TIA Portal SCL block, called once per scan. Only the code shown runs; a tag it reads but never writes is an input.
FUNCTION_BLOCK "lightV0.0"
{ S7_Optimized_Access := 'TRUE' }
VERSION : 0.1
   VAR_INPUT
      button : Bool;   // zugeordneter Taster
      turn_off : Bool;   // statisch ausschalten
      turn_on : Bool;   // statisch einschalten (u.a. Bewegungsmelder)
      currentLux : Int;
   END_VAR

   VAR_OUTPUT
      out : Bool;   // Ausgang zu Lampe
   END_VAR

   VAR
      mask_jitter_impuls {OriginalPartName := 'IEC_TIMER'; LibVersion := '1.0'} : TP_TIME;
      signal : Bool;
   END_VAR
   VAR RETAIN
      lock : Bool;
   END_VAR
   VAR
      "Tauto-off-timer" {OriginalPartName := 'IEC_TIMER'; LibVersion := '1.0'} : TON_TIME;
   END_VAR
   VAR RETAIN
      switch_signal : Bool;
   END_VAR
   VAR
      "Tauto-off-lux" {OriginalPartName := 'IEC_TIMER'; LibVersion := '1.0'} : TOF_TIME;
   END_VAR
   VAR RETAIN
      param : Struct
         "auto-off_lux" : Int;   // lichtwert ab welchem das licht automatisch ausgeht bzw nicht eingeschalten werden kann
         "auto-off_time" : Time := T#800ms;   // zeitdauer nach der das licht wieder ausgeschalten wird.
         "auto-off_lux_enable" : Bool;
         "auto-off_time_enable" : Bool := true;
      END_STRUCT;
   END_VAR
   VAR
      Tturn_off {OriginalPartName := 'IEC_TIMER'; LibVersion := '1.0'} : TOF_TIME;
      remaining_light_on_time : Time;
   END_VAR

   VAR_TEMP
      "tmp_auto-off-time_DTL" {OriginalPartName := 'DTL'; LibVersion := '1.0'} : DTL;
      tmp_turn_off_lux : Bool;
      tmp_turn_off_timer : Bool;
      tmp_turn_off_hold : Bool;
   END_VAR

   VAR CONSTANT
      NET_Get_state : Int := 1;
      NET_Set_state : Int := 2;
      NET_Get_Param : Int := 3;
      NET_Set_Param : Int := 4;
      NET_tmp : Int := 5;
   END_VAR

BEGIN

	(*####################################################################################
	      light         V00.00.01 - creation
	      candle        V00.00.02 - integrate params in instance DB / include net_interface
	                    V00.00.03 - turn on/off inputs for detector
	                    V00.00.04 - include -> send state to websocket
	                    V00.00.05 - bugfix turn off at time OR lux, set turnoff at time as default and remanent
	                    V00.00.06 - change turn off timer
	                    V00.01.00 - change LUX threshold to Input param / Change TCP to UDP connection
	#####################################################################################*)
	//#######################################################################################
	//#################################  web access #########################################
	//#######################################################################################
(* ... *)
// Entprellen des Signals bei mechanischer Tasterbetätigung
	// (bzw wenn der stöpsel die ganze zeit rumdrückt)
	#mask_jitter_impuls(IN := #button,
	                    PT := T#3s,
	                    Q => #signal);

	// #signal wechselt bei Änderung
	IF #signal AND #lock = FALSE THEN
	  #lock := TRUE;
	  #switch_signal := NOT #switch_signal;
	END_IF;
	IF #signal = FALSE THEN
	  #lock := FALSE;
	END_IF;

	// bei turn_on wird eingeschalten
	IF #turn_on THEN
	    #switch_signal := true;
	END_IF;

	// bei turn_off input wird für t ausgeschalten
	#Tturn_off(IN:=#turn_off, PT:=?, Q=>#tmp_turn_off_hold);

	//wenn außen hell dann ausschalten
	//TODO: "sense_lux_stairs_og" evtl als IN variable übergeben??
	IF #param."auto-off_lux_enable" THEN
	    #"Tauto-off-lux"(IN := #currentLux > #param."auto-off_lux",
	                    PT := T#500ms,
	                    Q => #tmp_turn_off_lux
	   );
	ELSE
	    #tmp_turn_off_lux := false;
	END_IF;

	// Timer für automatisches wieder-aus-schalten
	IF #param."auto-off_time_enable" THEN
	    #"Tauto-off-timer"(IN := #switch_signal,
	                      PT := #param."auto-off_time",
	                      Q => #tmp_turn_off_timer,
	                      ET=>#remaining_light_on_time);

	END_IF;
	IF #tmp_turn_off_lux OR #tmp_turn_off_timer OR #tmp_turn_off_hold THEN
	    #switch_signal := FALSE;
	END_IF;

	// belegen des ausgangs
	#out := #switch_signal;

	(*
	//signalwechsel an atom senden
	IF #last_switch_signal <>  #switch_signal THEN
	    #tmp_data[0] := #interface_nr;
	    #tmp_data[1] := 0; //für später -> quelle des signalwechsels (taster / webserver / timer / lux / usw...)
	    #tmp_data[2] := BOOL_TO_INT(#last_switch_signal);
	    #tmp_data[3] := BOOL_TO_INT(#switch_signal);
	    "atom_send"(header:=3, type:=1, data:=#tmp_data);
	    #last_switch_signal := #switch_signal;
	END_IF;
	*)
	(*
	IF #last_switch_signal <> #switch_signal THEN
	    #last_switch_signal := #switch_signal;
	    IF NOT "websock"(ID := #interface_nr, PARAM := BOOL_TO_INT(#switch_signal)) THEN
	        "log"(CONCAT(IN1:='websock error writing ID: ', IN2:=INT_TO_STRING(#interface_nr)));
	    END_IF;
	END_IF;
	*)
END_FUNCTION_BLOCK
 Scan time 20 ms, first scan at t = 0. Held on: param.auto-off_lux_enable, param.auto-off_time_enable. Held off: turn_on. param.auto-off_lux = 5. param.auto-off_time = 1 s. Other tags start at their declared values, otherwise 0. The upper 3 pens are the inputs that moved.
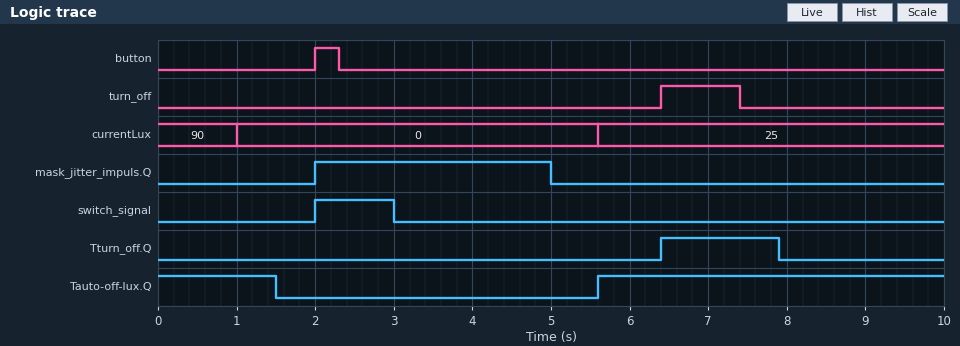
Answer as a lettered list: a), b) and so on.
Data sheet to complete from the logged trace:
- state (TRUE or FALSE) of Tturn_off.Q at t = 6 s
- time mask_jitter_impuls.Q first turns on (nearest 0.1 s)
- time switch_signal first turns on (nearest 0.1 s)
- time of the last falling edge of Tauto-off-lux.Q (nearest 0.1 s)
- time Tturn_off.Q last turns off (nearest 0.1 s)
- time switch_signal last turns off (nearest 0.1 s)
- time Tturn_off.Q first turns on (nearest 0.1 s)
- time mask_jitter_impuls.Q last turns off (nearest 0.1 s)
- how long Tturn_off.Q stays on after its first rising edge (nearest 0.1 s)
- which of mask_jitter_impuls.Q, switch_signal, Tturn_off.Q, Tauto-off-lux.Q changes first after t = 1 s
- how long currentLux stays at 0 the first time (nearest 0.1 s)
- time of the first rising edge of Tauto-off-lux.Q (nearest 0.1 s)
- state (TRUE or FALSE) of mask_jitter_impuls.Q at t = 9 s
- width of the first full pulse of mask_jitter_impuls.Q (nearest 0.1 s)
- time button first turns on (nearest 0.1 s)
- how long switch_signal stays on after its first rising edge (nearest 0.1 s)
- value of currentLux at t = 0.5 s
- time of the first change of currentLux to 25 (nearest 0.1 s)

a) FALSE
b) 2.0 s
c) 2.0 s
d) 1.5 s
e) 7.9 s
f) 3.0 s
g) 6.4 s
h) 5.0 s
i) 1.5 s
j) Tauto-off-lux.Q
k) 4.6 s
l) 5.6 s
m) FALSE
n) 3.0 s
o) 2.0 s
p) 1.0 s
q) 90
r) 5.6 s
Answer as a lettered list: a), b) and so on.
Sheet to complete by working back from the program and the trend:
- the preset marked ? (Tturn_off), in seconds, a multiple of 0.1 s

a) 0.5 s
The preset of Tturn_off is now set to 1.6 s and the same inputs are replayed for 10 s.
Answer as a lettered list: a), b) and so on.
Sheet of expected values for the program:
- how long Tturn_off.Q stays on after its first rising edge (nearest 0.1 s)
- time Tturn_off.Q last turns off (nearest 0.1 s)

a) 2.6 s
b) 9.0 s
